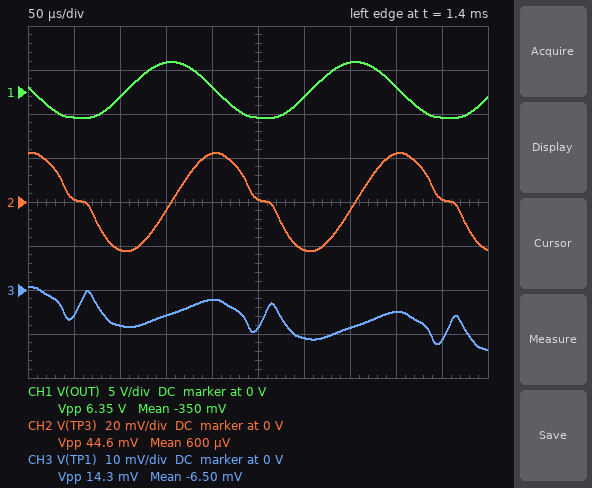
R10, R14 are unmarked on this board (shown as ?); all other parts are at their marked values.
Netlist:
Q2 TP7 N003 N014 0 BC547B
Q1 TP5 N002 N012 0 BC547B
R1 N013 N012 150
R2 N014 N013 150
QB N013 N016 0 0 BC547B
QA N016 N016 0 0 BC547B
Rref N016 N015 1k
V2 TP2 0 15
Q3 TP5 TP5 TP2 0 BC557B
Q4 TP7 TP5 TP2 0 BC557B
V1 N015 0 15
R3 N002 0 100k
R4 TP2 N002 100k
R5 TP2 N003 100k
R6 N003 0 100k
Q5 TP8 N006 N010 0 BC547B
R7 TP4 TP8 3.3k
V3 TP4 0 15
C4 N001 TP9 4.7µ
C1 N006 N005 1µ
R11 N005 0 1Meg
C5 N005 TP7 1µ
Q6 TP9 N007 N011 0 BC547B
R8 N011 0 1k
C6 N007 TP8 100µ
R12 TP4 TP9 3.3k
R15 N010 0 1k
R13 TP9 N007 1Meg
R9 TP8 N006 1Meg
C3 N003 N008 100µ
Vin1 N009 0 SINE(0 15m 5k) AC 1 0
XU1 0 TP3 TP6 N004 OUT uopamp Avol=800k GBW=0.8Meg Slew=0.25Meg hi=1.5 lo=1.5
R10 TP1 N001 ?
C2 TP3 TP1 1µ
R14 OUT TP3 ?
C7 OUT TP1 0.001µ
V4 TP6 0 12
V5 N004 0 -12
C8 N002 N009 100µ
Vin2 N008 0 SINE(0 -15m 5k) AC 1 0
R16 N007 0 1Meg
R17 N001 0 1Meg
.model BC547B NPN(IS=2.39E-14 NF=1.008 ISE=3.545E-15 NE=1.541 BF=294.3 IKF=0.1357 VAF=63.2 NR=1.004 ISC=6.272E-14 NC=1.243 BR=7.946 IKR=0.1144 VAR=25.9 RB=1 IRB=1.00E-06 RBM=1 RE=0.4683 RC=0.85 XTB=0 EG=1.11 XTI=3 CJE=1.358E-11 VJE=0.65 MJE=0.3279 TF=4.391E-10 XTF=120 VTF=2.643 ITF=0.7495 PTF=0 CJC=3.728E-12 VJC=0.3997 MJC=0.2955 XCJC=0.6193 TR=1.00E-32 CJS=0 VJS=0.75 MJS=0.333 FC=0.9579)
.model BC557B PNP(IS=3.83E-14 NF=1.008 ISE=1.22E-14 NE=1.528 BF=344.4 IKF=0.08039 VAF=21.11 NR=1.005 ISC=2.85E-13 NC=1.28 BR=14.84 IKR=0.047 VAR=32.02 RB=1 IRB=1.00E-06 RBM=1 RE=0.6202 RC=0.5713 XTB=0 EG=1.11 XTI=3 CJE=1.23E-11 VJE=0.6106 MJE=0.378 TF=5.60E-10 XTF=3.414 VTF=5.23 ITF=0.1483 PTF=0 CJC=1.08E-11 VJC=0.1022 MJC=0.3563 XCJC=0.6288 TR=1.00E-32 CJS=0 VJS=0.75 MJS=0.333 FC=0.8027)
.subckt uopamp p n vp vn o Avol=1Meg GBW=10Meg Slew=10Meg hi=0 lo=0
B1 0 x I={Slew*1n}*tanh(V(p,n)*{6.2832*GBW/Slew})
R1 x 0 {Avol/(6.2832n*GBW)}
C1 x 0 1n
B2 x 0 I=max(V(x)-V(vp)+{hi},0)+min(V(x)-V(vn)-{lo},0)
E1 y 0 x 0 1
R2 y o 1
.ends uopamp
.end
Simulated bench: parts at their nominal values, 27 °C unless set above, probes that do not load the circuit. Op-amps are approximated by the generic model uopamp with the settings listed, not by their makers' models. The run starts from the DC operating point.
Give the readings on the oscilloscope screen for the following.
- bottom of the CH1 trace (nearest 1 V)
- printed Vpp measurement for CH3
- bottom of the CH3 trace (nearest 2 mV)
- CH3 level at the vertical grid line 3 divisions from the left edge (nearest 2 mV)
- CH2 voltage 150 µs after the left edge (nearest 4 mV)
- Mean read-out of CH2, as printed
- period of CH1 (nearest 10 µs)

-3 V
14.3 mV
-14 mV
-6 mV
-4 mV
600 µV
200 µs
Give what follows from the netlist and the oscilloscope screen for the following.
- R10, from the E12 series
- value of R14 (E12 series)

6.8 kΩ
5.6 kΩ
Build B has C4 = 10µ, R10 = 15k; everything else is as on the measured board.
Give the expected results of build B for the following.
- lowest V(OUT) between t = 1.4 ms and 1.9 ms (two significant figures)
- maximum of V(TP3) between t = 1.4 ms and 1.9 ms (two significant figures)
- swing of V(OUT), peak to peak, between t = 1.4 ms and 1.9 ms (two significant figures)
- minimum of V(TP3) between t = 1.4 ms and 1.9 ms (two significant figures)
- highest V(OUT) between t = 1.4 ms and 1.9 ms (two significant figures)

-1.6 V
12 mV
3.5 V
-12 mV
1.9 V
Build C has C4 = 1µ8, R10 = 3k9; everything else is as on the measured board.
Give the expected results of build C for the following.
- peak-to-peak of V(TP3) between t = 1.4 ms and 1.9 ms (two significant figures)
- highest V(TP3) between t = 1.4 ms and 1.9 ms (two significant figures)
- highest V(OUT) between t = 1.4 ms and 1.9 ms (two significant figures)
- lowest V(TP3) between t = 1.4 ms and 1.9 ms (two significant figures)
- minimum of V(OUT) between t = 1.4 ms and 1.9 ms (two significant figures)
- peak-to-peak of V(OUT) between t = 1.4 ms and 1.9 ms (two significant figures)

68 mV
34 mV
4.8 V
-34 mV
-4.1 V
8.9 V
